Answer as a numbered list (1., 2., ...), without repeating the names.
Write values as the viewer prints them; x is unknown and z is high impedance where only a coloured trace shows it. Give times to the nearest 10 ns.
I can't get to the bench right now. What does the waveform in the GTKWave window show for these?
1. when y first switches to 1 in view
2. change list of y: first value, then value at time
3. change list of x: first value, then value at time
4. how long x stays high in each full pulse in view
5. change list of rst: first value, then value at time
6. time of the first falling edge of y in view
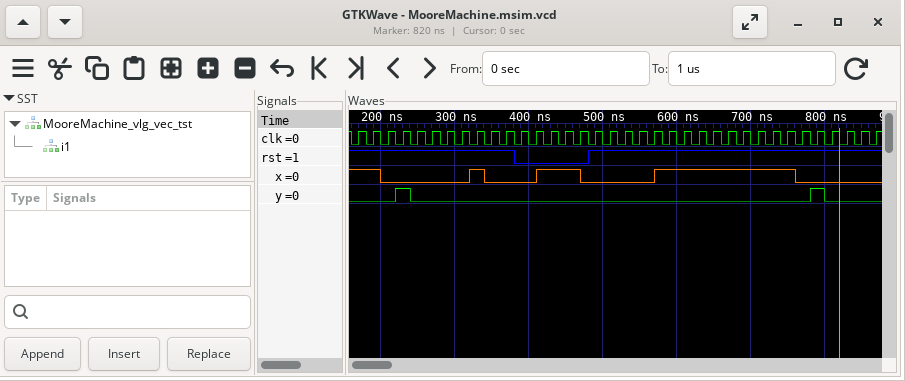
1. 220 ns
2. 0, 1 at 220 ns, 0 at 240 ns, 1 at 780 ns, 0 at 800 ns
3. 1, 0 at 200 ns, 1 at 320 ns, 0 at 340 ns, 1 at 410 ns, 0 at 470 ns, 1 at 570 ns, 0 at 760 ns
4. 20 ns, 60 ns, 190 ns
5. 1, 0 at 380 ns, 1 at 480 ns
6. 240 ns
